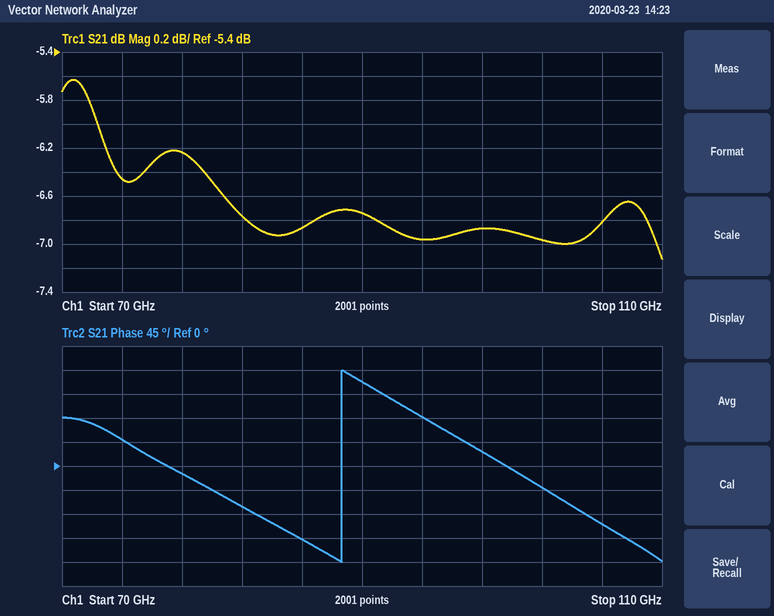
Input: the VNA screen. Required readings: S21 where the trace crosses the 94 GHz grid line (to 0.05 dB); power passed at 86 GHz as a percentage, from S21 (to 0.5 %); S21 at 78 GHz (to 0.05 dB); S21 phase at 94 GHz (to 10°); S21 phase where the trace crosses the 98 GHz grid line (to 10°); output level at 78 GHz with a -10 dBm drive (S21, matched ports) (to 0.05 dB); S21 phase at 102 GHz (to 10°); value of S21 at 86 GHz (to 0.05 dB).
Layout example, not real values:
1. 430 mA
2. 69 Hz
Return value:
1. -6.95 dB
2. 20.5 %
3. -6.25 dB
4. 90°
5. 30°
6. -16.25 dBm
7. -40°
8. -6.85 dB
